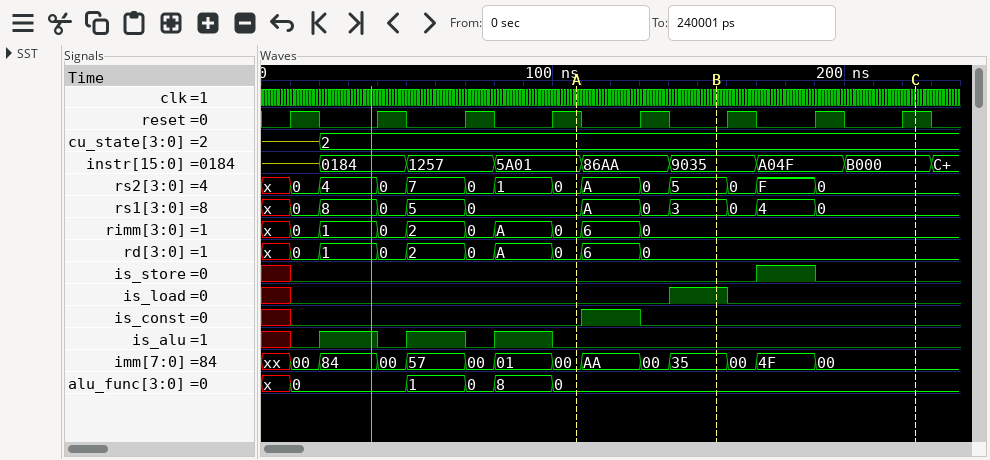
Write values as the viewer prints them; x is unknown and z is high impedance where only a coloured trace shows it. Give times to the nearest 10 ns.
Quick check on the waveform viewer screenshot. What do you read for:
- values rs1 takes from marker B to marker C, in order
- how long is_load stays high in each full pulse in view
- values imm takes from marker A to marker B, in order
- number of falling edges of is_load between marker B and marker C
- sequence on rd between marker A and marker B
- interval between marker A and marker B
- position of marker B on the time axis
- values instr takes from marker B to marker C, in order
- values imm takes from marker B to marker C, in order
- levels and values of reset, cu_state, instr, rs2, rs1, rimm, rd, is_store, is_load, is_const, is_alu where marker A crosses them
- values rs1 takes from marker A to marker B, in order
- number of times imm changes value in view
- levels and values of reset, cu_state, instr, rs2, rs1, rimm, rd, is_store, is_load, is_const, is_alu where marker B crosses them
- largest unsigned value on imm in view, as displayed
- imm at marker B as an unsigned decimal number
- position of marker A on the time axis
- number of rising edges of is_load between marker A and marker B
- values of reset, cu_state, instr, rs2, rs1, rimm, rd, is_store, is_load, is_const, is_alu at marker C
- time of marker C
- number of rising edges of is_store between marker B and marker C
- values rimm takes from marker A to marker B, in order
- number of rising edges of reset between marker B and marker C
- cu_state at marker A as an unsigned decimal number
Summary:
3, 0, 4, 0
20 ns
00, AA, 00, 35
1
0, 6, 0
50 ns
160 ns
9035, A04F, B000
35, 00, 4F, 00
reset=1, cu_state=2, instr=5A01, rs2=0, rs1=0, rimm=0, rd=0, is_store=0, is_load=0, is_const=0, is_alu=0
0, A, 0, 3
13
reset=0, cu_state=2, instr=9035, rs2=5, rs1=3, rimm=0, rd=0, is_store=0, is_load=1, is_const=0, is_alu=0
AA
53
110 ns
1
reset=1, cu_state=2, instr=B000, rs2=0, rs1=0, rimm=0, rd=0, is_store=0, is_load=0, is_const=0, is_alu=0
220 ns
1
0, 6, 0
3
2
